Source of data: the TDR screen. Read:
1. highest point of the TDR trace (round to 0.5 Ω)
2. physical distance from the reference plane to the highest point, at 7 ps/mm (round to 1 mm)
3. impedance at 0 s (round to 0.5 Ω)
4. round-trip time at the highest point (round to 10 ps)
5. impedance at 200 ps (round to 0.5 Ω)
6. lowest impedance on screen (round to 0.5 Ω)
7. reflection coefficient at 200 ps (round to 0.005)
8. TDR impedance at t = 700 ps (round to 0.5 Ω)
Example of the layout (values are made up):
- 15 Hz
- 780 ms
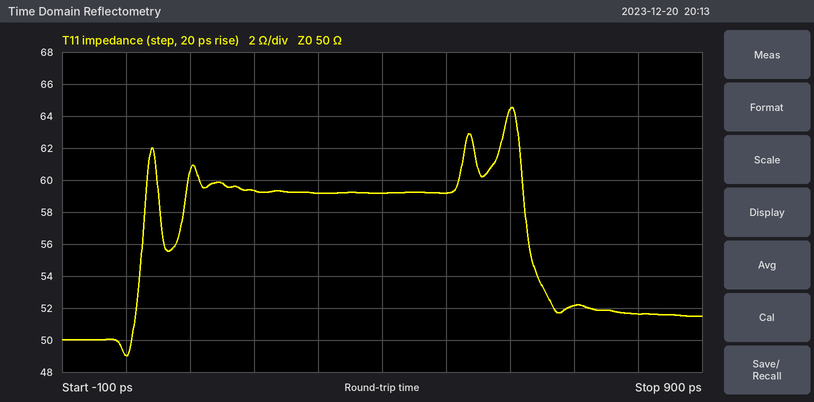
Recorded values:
- 64.5 Ω
- 43 mm
- 49.0 Ω
- 600 ps
- 59.5 Ω
- 49.0 Ω
- +0.085
- 52.0 Ω
